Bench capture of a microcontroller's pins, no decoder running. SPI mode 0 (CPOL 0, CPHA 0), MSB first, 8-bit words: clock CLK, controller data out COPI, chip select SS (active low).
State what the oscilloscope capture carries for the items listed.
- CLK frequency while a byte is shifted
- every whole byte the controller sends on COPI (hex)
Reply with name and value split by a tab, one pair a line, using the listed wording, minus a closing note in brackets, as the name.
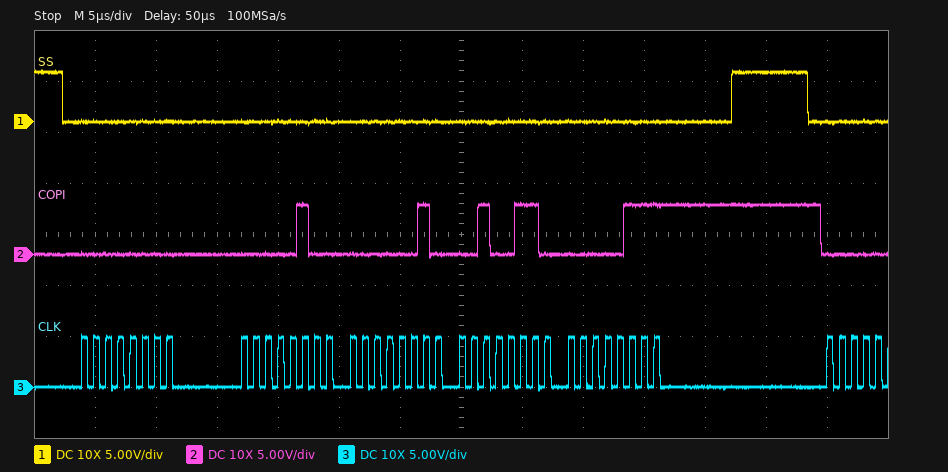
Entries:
CLK frequency while a byte is shifted	1 MHz
every whole byte the controller sends on COPI	0x00 0x04 0x02 0x26 0x07
